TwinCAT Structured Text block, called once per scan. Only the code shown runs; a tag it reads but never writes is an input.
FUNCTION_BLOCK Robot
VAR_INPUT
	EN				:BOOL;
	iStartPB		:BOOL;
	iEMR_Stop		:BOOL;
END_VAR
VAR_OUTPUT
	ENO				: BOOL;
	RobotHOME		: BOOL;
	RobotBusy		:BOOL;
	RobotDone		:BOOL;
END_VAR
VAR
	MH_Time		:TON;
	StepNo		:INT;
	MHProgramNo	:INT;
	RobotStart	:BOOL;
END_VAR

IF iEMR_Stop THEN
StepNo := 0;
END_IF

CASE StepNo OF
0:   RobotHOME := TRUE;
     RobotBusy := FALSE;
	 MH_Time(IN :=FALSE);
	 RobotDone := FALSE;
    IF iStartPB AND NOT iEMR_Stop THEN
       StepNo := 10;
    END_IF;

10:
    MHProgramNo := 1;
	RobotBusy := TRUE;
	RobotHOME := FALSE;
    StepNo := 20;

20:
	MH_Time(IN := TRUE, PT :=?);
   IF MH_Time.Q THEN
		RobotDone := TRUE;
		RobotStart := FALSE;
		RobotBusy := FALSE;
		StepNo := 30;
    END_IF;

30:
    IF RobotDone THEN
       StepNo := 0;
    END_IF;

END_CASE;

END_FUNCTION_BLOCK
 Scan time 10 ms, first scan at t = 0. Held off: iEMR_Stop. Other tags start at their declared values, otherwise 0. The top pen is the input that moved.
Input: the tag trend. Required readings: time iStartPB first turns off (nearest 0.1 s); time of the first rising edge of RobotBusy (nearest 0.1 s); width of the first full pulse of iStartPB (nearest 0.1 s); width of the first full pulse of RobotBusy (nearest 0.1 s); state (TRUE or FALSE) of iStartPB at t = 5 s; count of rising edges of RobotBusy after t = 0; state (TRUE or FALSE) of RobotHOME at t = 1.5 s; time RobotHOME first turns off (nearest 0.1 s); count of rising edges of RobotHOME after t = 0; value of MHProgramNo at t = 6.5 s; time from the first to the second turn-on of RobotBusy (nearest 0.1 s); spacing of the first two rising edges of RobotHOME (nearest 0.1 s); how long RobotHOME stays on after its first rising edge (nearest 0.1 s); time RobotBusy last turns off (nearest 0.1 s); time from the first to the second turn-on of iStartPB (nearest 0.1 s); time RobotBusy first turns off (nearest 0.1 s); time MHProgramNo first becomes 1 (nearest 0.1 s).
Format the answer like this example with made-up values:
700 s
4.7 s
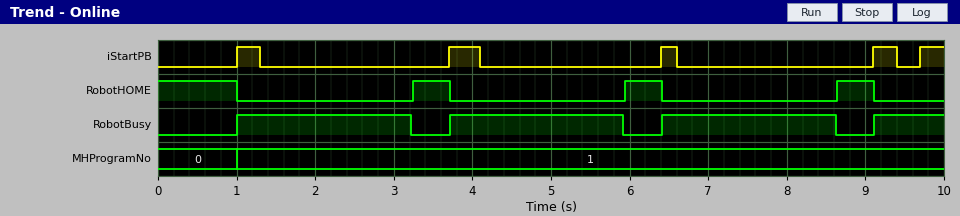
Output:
1.3 s
1.0 s
0.3 s
2.2 s
FALSE
4
FALSE
1.0 s
3
1
2.7 s
2.7 s
0.5 s
8.6 s
2.7 s
3.2 s
1.0 s
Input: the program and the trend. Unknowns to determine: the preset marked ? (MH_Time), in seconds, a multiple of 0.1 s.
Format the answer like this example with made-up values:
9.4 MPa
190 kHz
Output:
2.2 s
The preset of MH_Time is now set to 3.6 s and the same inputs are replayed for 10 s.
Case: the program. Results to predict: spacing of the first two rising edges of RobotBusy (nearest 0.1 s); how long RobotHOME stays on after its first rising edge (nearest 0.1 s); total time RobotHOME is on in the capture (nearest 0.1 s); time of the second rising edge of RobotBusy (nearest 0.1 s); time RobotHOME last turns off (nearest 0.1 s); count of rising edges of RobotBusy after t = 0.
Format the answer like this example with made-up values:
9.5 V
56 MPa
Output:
5.4 s
1.8 s
2.8 s
6.4 s
6.4 s
2
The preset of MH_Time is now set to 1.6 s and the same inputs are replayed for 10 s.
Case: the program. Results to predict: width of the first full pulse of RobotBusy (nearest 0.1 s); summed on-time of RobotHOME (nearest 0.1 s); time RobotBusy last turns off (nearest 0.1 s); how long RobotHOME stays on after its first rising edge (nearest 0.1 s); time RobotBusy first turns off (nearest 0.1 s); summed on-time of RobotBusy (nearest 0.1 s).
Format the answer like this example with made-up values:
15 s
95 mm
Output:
1.6 s
4.2 s
8.0 s
1.1 s
2.6 s
5.7 s
